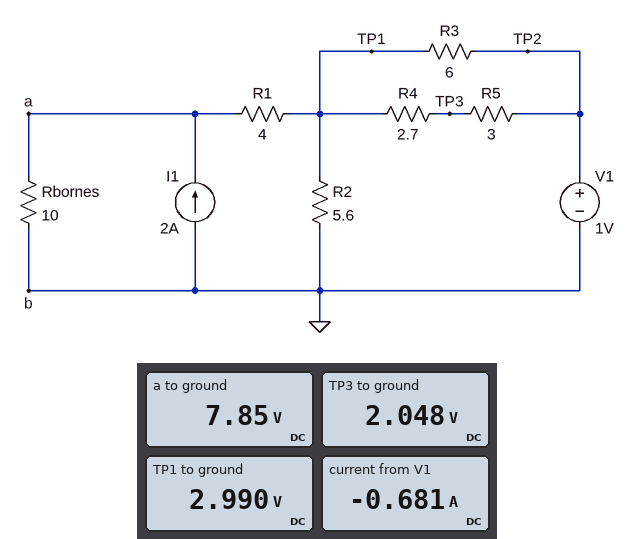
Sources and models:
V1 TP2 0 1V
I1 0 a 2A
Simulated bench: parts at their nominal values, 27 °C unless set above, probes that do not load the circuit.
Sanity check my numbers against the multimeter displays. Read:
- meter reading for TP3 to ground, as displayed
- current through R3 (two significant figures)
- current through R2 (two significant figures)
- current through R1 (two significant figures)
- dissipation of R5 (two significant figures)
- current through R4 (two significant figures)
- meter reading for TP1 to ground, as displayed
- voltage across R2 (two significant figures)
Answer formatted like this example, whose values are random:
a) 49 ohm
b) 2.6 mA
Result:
a) 2.048 V
b) 330 mA
c) 530 mA
d) 1.2 A
e) 370 mW
f) 350 mA
g) 2.990 V
h) 3.0 V
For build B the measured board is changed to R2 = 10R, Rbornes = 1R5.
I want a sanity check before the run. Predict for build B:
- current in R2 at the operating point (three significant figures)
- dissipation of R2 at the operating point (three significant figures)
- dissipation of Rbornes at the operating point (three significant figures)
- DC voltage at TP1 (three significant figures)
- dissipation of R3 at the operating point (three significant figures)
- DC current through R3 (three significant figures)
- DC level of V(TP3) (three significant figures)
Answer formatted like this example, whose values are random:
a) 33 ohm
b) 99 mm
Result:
a) 142 mA
b) 202 mW
c) 4.40 W
d) 1.42 V
e) 29.8 mW
f) 70.4 mA
g) 1.22 V
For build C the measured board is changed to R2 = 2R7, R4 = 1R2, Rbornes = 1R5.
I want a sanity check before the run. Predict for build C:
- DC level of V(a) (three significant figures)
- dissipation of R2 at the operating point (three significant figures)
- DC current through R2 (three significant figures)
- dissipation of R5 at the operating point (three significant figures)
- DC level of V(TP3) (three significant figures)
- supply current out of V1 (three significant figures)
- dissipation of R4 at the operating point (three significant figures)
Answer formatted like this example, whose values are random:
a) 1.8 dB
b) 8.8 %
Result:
a) 2.45 V
b) 365 mW
c) 368 mA
d) 8.42 µW
e) 995 mV
f) 2.85 mA
g) 3.37 µW
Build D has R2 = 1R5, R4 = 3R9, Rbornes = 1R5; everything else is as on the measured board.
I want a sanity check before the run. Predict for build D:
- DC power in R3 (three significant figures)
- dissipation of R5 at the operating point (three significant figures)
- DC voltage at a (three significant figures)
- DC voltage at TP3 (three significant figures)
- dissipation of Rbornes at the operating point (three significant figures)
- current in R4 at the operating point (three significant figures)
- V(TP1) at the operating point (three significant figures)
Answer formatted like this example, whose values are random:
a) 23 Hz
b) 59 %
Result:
a) 11.4 mW
b) 4.30 mW
c) 2.38 V
d) 886 mV
e) 3.79 W
f) 37.9 mA
g) 739 mV
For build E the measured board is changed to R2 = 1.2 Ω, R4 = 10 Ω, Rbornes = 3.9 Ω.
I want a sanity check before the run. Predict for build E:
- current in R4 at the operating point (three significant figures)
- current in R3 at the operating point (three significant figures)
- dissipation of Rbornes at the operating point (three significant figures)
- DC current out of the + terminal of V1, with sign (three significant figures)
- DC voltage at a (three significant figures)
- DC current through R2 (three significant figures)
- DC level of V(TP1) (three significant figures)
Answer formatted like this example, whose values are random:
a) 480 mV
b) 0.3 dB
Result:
a) 1.75 mA
b) 3.80 mA
c) 5.09 W
d) -5.55 mA
e) 4.45 V
f) 852 mA
g) 1.02 V
